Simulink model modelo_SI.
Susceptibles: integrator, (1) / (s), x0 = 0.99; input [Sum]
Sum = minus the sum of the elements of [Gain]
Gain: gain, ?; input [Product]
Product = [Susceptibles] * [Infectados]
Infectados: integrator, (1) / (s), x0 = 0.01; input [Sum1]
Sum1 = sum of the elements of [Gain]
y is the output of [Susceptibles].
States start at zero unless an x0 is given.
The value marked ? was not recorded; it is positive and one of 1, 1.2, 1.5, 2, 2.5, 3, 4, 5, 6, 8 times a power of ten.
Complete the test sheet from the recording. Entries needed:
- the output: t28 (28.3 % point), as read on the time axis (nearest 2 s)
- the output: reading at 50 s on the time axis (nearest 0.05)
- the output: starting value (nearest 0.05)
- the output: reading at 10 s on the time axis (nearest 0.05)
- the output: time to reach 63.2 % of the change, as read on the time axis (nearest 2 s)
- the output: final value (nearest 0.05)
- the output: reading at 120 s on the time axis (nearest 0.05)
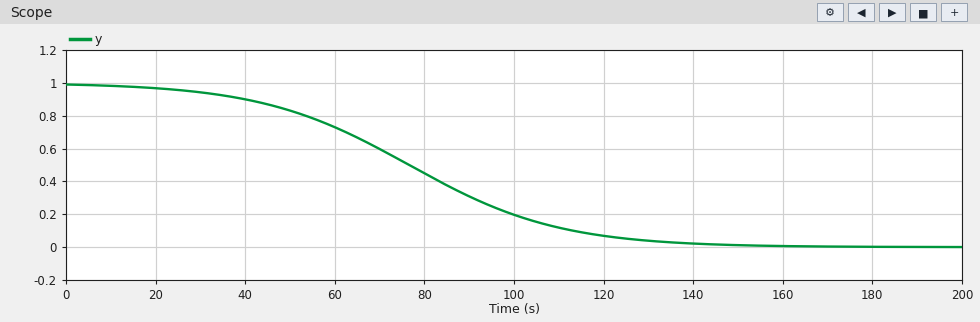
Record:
62 s
0.85
1.00
1.00
86 s
0.00
0.05
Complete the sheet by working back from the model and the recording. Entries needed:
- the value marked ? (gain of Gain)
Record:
0.06
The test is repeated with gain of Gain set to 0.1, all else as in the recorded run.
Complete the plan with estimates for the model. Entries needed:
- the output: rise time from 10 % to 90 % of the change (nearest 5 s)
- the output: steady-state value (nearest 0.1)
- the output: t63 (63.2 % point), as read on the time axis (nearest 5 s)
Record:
45 s
0.0
50 s
